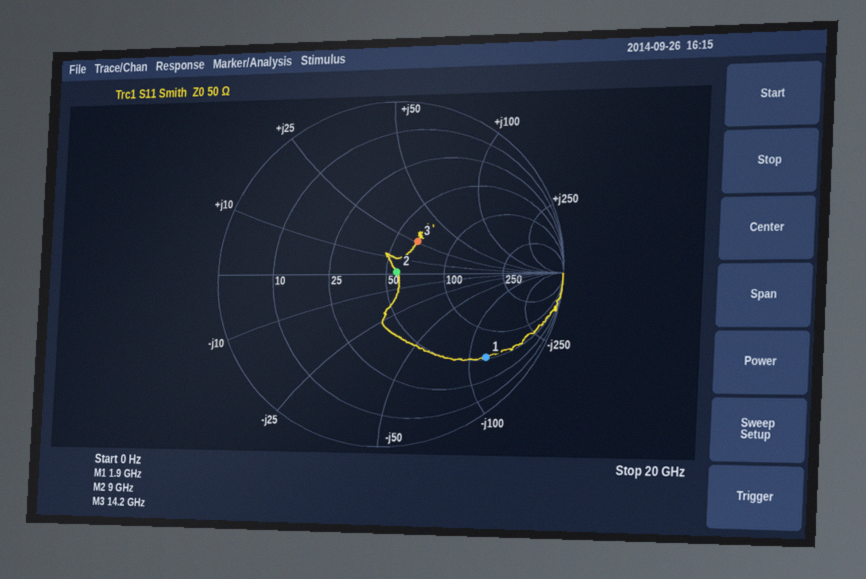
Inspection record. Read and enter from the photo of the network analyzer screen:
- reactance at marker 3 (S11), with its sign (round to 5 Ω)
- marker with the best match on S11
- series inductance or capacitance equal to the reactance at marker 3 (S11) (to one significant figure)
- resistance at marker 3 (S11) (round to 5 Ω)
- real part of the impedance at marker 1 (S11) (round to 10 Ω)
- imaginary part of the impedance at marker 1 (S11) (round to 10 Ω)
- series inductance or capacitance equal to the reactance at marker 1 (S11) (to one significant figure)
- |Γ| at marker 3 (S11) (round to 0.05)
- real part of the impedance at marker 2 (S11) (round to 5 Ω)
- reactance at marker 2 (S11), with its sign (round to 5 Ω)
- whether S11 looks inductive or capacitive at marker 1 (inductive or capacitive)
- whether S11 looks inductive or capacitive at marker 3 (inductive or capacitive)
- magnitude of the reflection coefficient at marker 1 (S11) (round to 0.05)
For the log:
+25 Ω
marker 2
300 pH
65 Ω
50 Ω
-120 Ω
700 fF
0.25
55 Ω
0 Ω
capacitive
inductive
0.75
